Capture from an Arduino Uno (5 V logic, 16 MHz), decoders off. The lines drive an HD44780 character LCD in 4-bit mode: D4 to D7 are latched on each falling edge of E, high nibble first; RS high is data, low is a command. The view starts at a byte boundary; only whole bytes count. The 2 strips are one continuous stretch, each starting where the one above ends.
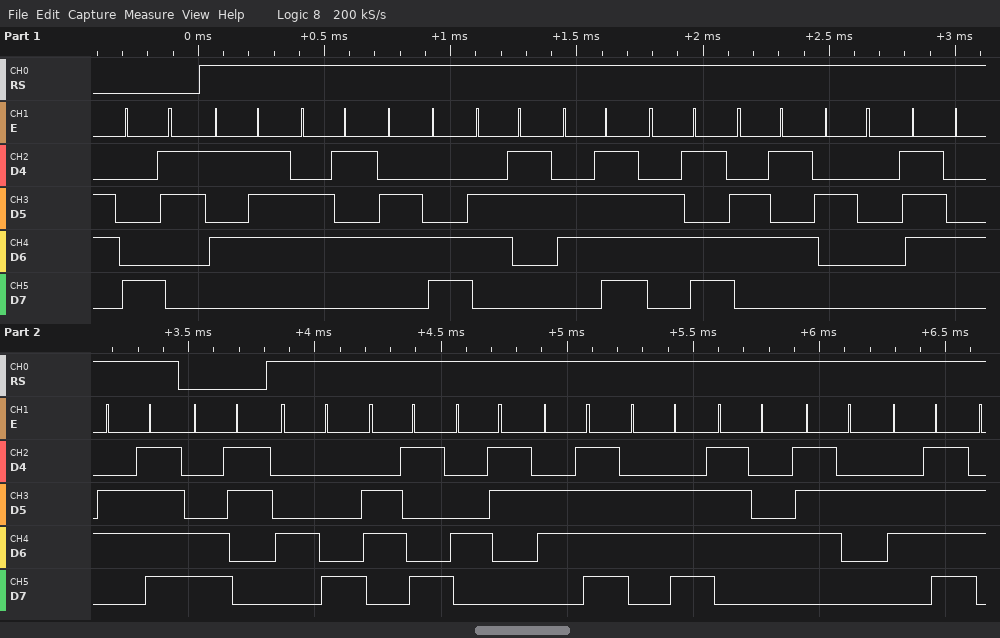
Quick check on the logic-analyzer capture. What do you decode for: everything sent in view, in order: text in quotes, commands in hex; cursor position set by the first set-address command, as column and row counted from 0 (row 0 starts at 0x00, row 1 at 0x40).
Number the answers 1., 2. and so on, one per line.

1. 0x83 "Welcome to" 0xC3 "HiContro"
2. column 3, row 0
